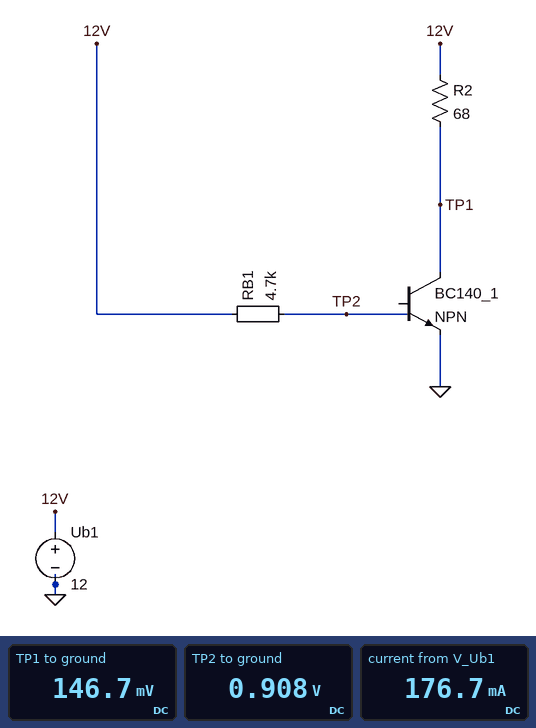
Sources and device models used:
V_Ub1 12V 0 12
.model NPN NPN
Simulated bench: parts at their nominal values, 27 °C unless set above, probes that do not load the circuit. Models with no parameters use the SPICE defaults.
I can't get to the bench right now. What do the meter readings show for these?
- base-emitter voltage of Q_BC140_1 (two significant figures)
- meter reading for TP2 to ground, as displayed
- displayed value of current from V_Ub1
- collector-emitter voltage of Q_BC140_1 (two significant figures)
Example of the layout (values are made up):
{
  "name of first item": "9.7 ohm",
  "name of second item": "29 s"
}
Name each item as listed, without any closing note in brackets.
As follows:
{
  "base-emitter voltage of Q_BC140_1": "910 mV",
  "meter reading for TP2 to ground, as displayed": "0.908 V",
  "displayed value of current from V_Ub1": "176.7 mA",
  "collector-emitter voltage of Q_BC140_1": "150 mV"
}
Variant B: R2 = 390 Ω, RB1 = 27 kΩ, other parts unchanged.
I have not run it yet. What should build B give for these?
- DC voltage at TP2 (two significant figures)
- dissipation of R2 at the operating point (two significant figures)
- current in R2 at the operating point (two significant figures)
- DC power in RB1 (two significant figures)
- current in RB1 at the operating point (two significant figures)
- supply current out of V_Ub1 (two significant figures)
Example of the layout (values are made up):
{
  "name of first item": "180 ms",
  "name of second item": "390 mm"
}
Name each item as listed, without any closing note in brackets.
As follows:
{
  "DC voltage at TP2": "860 mV",
  "dissipation of R2 at the operating point": "360 mW",
  "current in R2 at the operating point": "30 mA",
  "DC power in RB1": "4.6 mW",
  "current in RB1 at the operating point": "410 µA",
  "supply current out of V_Ub1": "31 mA"
}
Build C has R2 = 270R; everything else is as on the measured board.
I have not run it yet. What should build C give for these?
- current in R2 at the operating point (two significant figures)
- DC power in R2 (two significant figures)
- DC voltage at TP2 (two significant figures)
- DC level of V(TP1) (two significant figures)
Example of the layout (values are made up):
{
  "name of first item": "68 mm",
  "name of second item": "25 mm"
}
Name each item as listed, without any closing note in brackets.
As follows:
{
  "current in R2 at the operating point": "44 mA",
  "DC power in R2": "530 mW",
  "DC voltage at TP2": "870 mV",
  "DC level of V(TP1)": "84 mV"
}
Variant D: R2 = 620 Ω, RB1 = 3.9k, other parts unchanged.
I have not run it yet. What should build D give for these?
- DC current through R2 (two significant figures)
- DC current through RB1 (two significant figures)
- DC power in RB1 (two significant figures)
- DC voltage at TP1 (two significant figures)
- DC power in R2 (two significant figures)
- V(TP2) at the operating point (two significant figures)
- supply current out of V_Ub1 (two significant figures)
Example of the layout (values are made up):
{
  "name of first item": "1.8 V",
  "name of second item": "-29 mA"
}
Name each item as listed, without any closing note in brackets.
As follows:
{
  "DC current through R2": "19 mA",
  "DC current through RB1": "2.9 mA",
  "DC power in RB1": "32 mW",
  "DC voltage at TP1": "58 mV",
  "DC power in R2": "230 mW",
  "V(TP2) at the operating point": "860 mV",
  "supply current out of V_Ub1": "22 mA"
}
